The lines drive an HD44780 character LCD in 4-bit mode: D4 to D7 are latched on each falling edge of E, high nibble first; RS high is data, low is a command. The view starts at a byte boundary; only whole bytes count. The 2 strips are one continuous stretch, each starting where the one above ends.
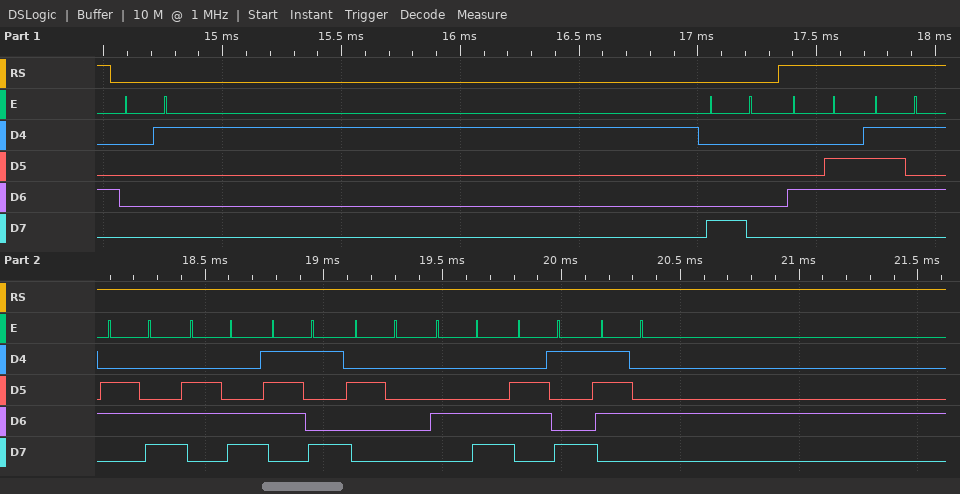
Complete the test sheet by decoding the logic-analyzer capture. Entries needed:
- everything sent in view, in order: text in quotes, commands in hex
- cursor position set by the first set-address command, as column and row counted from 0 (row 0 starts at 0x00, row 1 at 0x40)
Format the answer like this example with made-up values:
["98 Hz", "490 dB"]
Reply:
["0x01 0x80 \"Fully Lit\"", "column 0, row 0"]
